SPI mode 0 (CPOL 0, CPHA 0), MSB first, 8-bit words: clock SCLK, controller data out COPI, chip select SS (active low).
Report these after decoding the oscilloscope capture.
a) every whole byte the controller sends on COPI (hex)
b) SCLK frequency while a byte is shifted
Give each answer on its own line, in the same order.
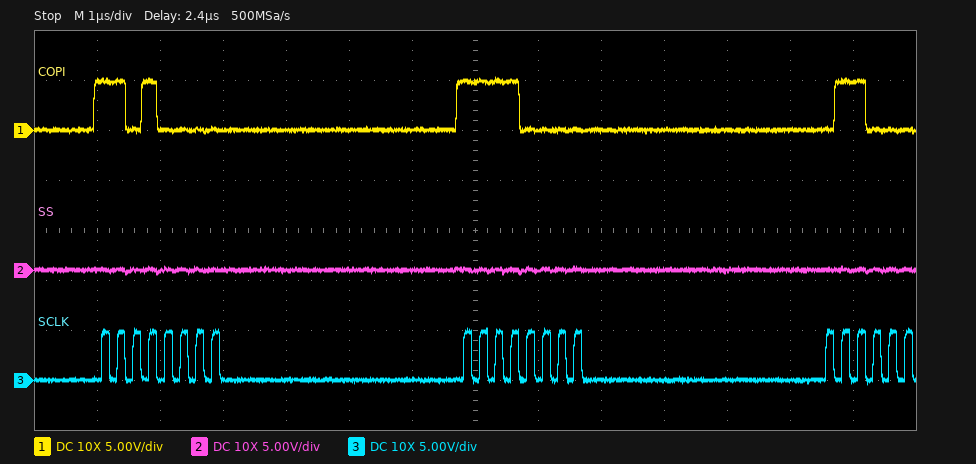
D0 F0
4 MHz
